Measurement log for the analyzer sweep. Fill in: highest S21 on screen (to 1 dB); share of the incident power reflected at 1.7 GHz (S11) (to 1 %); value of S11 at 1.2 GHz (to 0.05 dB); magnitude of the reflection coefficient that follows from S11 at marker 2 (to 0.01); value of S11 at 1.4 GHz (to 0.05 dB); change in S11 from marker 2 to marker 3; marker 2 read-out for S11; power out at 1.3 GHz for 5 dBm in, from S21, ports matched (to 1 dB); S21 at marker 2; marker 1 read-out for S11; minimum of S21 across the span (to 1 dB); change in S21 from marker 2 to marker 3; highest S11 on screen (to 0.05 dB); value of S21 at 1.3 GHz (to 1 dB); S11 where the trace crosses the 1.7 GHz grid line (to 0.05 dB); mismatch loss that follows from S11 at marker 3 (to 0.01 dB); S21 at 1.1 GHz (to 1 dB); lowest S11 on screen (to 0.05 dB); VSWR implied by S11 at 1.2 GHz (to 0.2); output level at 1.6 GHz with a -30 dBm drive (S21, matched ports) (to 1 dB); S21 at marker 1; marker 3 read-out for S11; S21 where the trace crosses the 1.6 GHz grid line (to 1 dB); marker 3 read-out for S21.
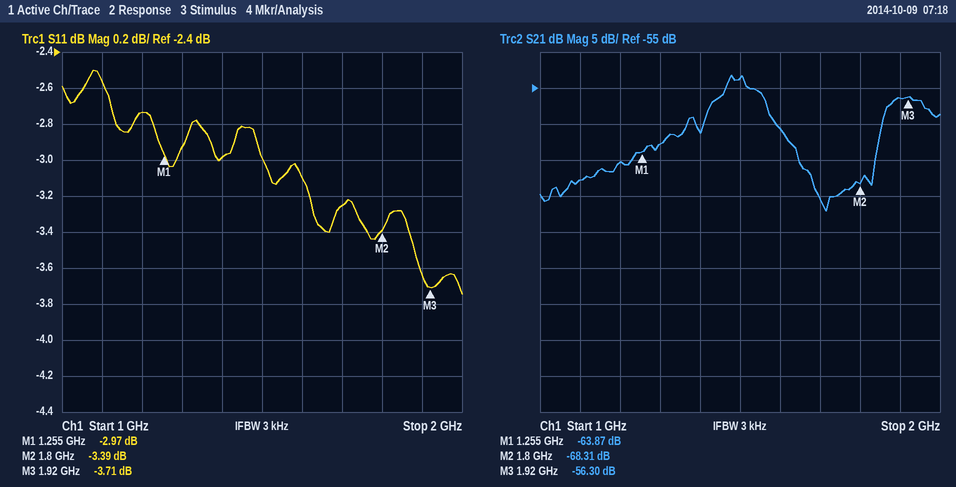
-53 dB
47 %
-2.75 dB
0.68
-3.00 dB
-0.32 dB
-3.39 dB
-58 dBm
-68.31 dB
-2.97 dB
-72 dB
12.01 dB
-2.50 dB
-63 dB
-3.25 dB
2.41 dB
-68 dB
-3.75 dB
6.4
-91 dBm
-63.87 dB
-3.71 dB
-61 dB
-56.30 dB
